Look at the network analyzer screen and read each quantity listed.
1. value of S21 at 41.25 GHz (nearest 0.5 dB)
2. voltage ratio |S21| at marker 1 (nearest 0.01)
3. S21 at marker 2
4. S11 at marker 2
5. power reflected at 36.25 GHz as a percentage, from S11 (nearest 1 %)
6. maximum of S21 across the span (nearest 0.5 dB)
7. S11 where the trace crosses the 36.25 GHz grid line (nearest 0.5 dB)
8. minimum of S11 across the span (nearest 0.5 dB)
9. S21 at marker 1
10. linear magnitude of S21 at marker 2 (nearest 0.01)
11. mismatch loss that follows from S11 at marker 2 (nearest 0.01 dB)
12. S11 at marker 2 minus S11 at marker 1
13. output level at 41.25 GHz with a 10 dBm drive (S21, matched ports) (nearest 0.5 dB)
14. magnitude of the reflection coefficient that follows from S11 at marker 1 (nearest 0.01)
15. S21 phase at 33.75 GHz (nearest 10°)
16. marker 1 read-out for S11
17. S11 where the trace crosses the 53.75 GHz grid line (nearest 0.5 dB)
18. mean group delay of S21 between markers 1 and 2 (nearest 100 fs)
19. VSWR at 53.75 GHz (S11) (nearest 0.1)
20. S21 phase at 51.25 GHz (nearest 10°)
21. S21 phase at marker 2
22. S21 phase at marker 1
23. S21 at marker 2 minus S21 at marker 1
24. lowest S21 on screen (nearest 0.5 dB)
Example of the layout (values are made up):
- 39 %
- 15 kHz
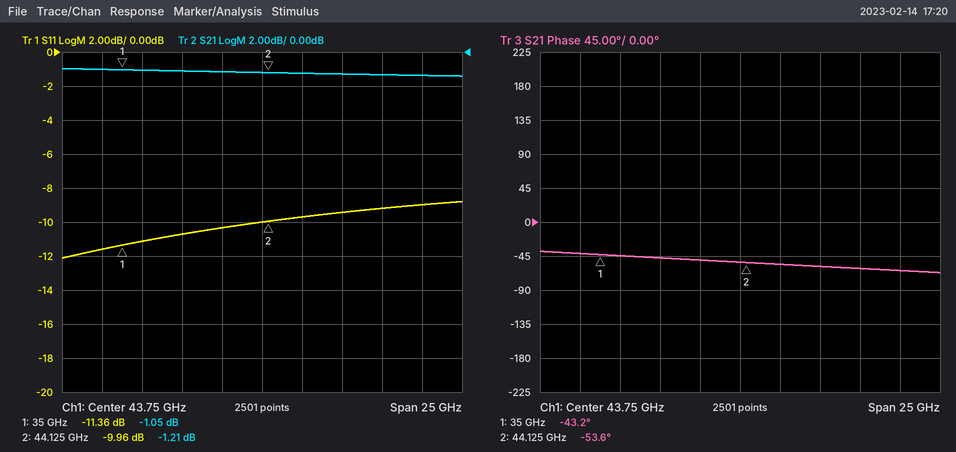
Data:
- -1.0 dB
- 0.89
- -1.21 dB
- -9.96 dB
- 8 %
- -1.0 dB
- -11.0 dB
- -12.0 dB
- -1.05 dB
- 0.87
- 0.46 dB
- 1.40 dB
- 9.0 dBm
- 0.27
- -40°
- -11.36 dB
- -9.0 dB
- 3.2 ps
- 2.1
- -60°
- -53.6°
- -43.2°
- -0.16 dB
- -1.5 dB
